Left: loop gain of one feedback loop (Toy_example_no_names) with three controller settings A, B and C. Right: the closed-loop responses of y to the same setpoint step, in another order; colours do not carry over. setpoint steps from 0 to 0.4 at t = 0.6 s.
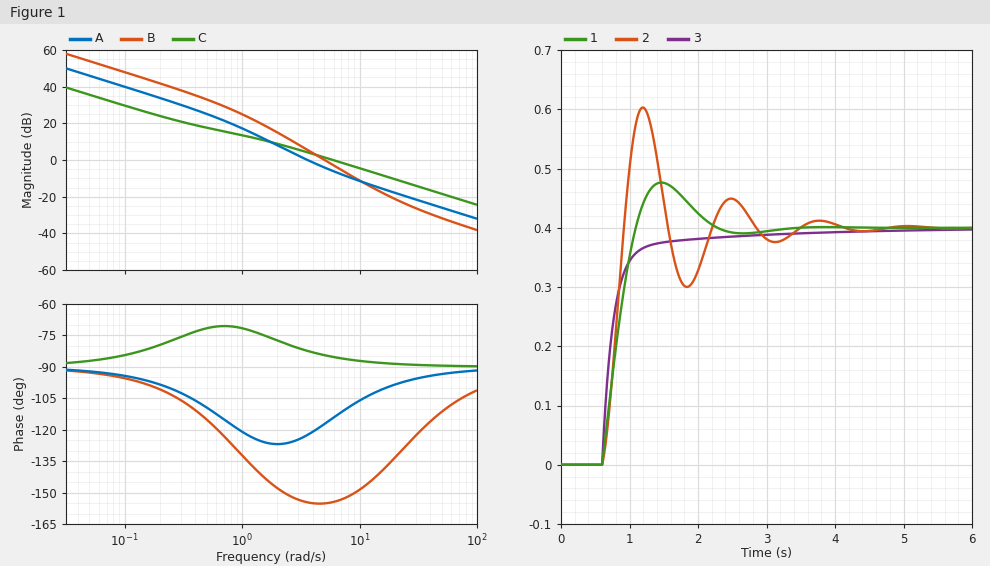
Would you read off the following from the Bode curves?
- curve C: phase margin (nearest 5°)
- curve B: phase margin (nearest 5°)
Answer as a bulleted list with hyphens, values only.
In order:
- 95°
- 25°
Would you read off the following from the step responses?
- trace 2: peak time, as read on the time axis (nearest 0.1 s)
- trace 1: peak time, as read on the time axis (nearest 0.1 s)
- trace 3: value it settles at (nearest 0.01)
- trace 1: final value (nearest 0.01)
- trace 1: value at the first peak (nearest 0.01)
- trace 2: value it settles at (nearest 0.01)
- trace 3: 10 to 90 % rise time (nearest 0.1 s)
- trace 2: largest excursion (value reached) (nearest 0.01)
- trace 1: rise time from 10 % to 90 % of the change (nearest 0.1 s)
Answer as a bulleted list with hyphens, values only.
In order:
- 1.2 s
- 1.5 s
- 0.40
- 0.40
- 0.48
- 0.40
- 0.5 s
- 0.60
- 0.4 s
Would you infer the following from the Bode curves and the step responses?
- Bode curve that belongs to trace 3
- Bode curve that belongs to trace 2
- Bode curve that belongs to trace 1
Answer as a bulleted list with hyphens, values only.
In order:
- C
- B
- A
